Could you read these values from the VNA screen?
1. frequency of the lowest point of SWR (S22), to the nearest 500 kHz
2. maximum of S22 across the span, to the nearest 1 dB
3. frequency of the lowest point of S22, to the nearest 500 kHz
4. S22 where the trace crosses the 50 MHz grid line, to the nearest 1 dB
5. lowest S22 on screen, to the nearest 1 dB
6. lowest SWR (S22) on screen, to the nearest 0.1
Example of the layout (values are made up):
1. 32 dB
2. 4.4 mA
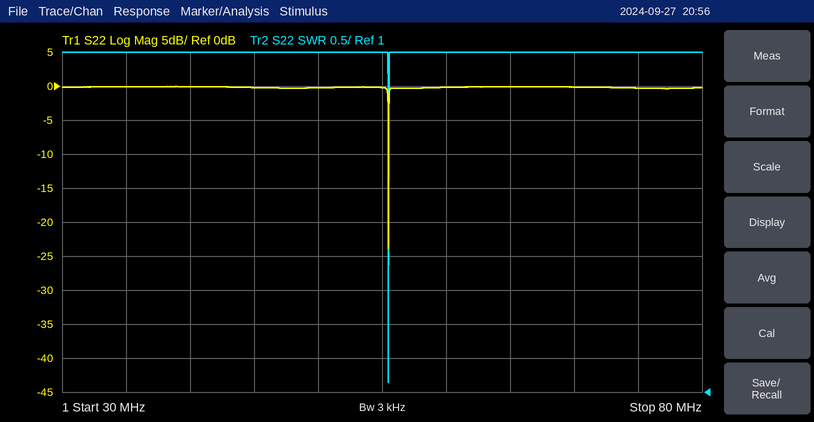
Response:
1. 55.5 MHz
2. 0 dB
3. 55.5 MHz
4. 0 dB
5. -24 dB
6. 1.1
